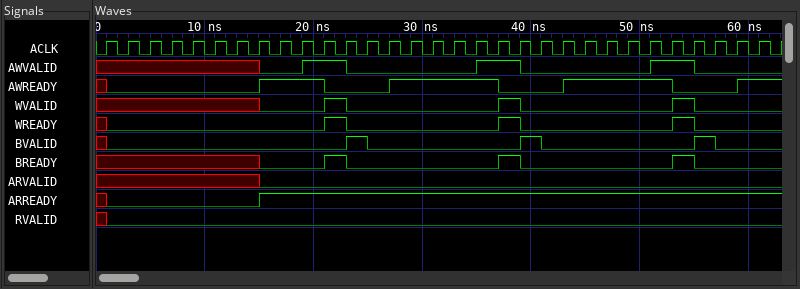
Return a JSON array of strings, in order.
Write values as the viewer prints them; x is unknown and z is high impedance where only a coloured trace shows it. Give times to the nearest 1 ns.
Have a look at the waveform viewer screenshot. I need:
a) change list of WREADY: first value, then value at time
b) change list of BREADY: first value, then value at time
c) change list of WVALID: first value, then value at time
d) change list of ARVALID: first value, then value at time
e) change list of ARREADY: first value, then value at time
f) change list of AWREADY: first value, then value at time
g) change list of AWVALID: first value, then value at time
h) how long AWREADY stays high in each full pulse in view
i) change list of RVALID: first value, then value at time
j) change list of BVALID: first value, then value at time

["x, 0 at 1 ns, 1 at 21 ns, 0 at 23 ns, 1 at 37 ns, 0 at 39 ns, 1 at 53 ns, 0 at 55 ns", "x, 0 at 15 ns, 1 at 21 ns, 0 at 23 ns, 1 at 37 ns, 0 at 39 ns, 1 at 53 ns, 0 at 55 ns", "x, 0 at 15 ns, 1 at 21 ns, 0 at 23 ns, 1 at 37 ns, 0 at 39 ns, 1 at 53 ns, 0 at 55 ns", "x, 0 at 15 ns", "x, 0 at 1 ns, 1 at 15 ns", "x, 0 at 1 ns, 1 at 15 ns, 0 at 21 ns, 1 at 27 ns, 0 at 37 ns, 1 at 43 ns, 0 at 53 ns, 1 at 59 ns", "x, 0 at 15 ns, 1 at 19 ns, 0 at 23 ns, 1 at 35 ns, 0 at 39 ns, 1 at 51 ns, 0 at 55 ns", "6 ns, 10 ns, 10 ns", "x, 0 at 1 ns", "x, 0 at 1 ns, 1 at 23 ns, 0 at 25 ns, 1 at 39 ns, 0 at 41 ns, 1 at 55 ns, 0 at 57 ns"]
